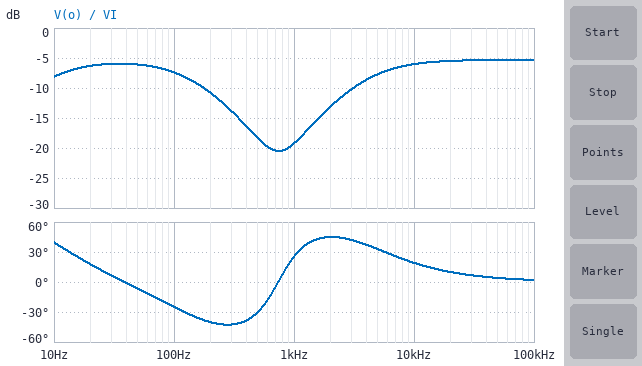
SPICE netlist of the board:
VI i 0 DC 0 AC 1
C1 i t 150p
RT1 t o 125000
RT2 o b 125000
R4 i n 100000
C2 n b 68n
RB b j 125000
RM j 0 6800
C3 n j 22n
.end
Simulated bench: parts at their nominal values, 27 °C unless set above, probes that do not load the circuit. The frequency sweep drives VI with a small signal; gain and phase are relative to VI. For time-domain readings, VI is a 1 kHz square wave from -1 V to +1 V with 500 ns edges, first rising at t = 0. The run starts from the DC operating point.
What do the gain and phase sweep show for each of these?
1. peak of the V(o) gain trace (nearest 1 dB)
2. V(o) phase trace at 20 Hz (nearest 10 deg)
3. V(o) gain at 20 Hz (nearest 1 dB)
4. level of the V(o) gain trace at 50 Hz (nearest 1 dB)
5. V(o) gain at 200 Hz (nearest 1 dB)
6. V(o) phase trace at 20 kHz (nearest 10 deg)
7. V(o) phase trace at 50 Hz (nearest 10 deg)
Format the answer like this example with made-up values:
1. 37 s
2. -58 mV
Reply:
1. -5 dB
2. 20 deg
3. -6 dB
4. -6 dB
5. -11 dB
6. 10 deg
7. -10 deg
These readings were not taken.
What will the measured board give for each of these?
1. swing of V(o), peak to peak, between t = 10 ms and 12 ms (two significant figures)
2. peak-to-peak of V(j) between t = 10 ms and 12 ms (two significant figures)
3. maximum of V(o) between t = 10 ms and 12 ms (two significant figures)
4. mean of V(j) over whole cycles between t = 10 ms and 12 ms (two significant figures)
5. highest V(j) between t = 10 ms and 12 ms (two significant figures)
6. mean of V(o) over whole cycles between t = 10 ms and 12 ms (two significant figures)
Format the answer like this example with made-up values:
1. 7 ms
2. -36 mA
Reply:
1. 1.9 V
2. 240 mV
3. 1.2 V
4. 18 mV
5. 140 mV
6. 300 mV
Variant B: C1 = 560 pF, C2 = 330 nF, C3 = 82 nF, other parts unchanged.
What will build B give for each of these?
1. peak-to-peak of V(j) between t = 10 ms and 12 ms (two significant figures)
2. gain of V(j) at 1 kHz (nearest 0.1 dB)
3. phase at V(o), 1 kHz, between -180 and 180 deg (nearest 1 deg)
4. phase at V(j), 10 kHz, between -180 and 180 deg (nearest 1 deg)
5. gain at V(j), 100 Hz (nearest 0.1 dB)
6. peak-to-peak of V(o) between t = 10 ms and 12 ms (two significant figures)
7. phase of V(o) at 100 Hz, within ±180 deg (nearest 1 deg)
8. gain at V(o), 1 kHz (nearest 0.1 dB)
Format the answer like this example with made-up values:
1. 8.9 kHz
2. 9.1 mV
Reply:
1. 220 mV
2. -22.5 dB
3. 39 deg
4. 2 deg
5. -24.3 dB
6. 1.9 V
7. -41 deg
8. -9.0 dB
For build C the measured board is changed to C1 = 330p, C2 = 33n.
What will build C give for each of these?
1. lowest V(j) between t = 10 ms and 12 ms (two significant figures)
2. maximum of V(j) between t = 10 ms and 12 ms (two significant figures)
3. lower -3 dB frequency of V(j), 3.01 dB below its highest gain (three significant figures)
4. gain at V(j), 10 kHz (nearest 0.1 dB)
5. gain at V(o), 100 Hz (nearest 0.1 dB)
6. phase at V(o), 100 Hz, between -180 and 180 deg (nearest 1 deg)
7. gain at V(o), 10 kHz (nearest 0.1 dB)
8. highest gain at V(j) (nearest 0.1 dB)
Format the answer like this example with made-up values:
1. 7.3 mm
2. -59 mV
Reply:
1. -110 mV
2. 130 mV
3. 375 Hz
4. -21.3 dB
5. -7.8 dB
6. -16 deg
7. -5.5 dB
8. -21.2 dB
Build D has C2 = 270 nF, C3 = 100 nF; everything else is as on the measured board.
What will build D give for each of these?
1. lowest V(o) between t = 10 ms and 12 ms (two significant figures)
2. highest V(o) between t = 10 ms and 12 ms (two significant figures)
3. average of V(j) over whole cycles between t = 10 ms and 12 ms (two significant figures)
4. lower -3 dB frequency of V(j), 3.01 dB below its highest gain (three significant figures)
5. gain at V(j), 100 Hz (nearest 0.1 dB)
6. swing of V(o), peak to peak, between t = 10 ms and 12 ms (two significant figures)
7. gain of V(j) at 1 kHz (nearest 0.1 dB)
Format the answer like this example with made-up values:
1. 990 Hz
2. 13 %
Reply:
1. -570 mV
2. 1.4 V
3. 33 mV
4. 90.4 Hz
5. -24.2 dB
6. 2.0 V
7. -23.7 dB
